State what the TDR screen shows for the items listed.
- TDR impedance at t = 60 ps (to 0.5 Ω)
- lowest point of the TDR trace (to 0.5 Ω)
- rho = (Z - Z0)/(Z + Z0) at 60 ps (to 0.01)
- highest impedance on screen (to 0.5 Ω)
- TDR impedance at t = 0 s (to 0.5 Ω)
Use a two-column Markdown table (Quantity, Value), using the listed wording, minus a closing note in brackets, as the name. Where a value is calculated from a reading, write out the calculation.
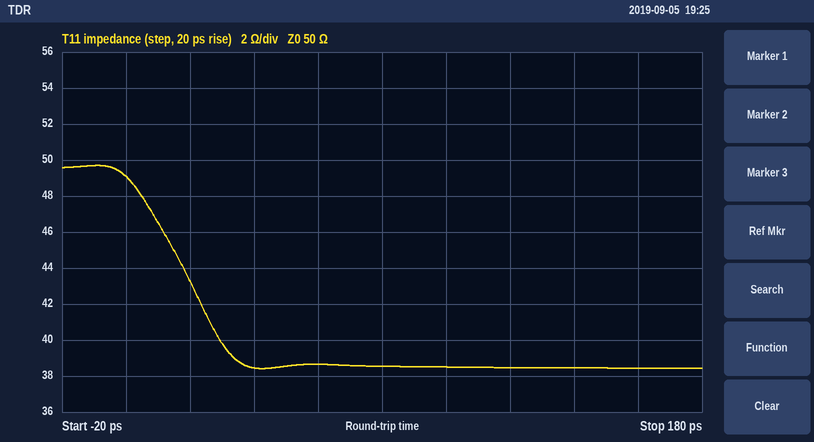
| Quantity | Value |
|---|---|
| TDR impedance at t = 60 ps | 38.5 Ω |
| lowest point of the TDR trace | 38.5 Ω |
| rho = (Z - Z0)/(Z + Z0) at 60 ps | (38.5 − 50)/(38.5 + 50) ≈ -0.13 |
| highest impedance on screen | 49.5 Ω |
| TDR impedance at t = 0 s | 49.0 Ω |
